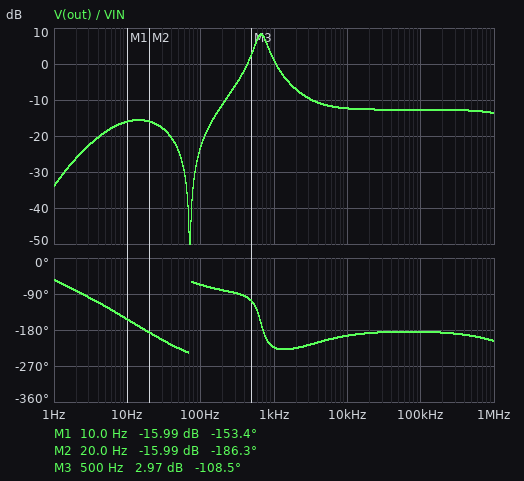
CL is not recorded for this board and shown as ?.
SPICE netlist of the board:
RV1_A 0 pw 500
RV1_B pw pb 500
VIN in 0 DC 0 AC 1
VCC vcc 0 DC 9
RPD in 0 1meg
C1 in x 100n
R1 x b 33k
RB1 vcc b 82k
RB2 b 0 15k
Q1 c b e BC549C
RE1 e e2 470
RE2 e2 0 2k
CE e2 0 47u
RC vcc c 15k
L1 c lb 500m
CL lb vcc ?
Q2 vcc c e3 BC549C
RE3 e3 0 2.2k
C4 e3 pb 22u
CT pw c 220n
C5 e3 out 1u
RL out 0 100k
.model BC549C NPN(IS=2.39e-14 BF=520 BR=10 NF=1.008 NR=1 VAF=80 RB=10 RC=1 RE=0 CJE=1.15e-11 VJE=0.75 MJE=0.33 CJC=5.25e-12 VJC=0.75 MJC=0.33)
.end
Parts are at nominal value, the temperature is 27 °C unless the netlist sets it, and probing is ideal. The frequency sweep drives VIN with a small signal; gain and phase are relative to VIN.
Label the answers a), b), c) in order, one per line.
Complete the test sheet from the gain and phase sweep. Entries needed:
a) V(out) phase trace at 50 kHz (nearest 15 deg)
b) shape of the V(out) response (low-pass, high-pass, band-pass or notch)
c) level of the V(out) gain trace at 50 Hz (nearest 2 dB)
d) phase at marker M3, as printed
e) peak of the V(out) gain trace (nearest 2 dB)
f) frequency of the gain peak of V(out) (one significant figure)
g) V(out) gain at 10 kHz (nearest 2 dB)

a) -180 deg
b) band-pass
c) -24 dB
d) -108.5 deg
e) 8 dB
f) 700 Hz
g) -12 dB
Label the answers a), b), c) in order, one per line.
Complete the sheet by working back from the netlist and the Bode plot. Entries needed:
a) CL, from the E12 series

a) 10 µF
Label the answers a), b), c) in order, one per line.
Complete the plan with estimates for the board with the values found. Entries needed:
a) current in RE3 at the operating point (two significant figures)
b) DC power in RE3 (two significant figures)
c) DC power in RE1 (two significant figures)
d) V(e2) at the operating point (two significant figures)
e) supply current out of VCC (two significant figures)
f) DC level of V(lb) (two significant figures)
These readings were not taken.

a) 1.6 mA
b) 5.9 mW
c) 47 µW
d) 630 mV
e) 2.0 mA
f) 4.2 V
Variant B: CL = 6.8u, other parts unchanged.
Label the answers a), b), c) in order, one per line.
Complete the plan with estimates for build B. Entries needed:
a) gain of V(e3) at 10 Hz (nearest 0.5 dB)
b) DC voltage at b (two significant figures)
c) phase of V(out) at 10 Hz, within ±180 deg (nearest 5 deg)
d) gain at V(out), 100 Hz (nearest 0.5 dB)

a) -12.5 dB
b) 1.4 V
c) -150 deg
d) -29.0 dB
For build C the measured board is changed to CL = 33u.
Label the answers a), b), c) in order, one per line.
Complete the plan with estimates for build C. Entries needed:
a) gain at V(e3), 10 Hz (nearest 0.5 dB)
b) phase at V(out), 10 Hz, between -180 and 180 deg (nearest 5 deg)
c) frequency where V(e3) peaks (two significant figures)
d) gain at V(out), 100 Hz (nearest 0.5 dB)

a) -26.5 dB
b) -160 deg
c) 660 Hz
d) -18.5 dB
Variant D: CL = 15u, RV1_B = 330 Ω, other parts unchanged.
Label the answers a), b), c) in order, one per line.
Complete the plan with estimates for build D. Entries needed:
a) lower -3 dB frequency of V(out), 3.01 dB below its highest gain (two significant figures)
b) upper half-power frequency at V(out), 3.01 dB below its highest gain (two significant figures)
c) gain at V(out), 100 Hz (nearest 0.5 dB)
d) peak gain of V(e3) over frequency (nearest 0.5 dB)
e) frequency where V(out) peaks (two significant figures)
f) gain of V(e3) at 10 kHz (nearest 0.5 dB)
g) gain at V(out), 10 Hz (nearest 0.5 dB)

a) 610 Hz
b) 900 Hz
c) -20.5 dB
d) 9.0 dB
e) 740 Hz
f) -12.0 dB
g) -19.5 dB
